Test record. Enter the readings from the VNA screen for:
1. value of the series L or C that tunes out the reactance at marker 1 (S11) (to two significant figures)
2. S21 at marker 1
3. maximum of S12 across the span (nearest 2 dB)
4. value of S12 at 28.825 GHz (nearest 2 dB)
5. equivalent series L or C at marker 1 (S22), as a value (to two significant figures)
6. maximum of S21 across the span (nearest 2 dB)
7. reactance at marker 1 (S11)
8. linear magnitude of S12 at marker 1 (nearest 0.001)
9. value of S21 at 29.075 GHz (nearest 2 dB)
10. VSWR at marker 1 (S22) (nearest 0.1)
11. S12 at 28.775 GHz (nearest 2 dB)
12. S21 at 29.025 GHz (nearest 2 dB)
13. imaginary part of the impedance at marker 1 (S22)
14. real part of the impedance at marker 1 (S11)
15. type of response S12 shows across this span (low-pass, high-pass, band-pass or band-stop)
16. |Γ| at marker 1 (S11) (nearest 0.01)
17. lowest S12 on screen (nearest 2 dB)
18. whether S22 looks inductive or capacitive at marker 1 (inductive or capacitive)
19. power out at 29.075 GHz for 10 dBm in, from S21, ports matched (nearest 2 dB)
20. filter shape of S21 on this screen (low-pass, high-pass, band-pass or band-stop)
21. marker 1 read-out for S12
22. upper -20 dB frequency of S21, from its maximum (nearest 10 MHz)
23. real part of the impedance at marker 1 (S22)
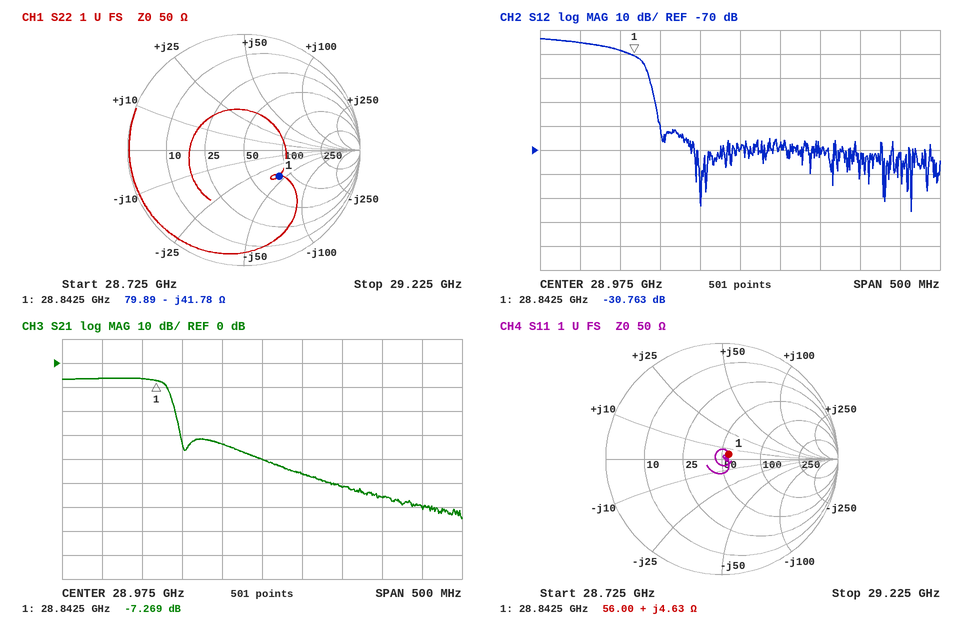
1.2 pF
-7.269 dB
-24 dB
-28 dB
130 fF
-6 dB
+4.63 Ω
0.029
-52 dB
2.2
-26 dB
-46 dB
-41.78 Ω
56.00 Ω
low-pass
0.07
-96 dB
capacitive
-42 dBm
low-pass
-30.763 dB
28.87 GHz
79.89 Ω
